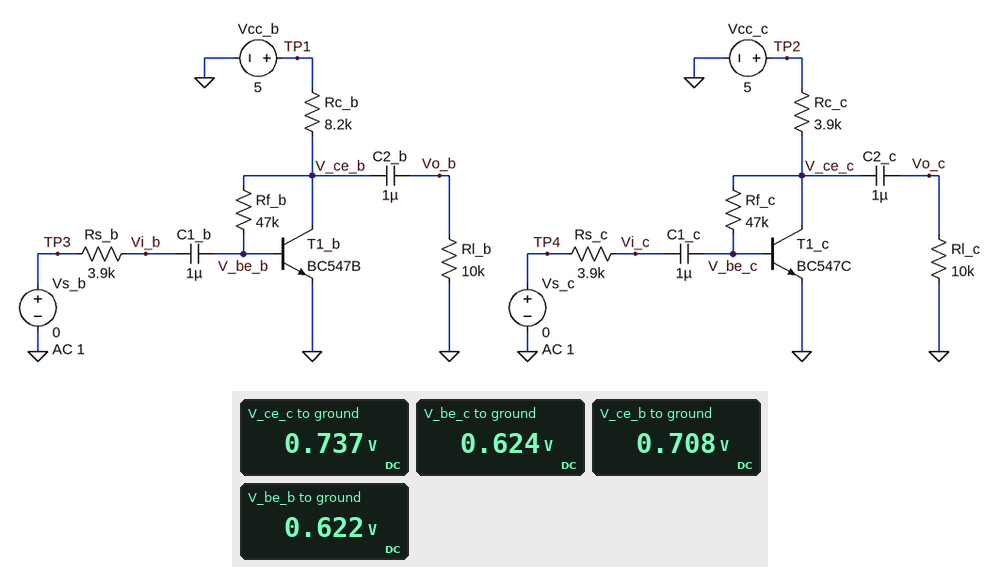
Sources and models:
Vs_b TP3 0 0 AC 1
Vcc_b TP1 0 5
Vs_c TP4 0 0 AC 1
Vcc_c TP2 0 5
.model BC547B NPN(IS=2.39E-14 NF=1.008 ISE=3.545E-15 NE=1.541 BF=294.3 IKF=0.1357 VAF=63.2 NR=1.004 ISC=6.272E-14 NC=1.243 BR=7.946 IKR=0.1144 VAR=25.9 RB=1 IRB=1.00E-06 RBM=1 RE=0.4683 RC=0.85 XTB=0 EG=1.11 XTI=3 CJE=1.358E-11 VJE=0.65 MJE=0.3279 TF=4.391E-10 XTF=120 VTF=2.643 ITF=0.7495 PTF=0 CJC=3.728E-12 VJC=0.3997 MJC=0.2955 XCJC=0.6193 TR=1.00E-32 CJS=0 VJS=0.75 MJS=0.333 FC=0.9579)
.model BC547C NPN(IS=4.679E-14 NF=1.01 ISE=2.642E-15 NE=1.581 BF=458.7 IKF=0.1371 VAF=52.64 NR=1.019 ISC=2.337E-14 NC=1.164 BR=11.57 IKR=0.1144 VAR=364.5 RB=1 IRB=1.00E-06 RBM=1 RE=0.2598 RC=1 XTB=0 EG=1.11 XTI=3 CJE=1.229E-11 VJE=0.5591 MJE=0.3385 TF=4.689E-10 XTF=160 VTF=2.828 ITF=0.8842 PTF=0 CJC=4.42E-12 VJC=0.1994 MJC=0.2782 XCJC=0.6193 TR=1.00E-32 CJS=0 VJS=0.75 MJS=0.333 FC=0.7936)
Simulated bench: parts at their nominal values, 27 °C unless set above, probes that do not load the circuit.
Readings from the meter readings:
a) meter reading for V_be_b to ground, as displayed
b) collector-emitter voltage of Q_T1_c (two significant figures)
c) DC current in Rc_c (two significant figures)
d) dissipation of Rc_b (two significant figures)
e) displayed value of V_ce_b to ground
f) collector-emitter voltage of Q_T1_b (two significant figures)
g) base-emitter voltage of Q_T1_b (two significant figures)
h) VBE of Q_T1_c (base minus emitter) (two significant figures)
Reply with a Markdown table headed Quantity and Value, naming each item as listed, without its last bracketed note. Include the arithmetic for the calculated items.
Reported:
| Quantity | Value |
|---|---|
| meter reading for V_be_b to ground, as displayed | 0.622 V |
| collector-emitter voltage of Q_T1_c | 737 mV = 740 mV |
| DC current in Rc_c | (5 V - 737 mV) / 3.9 kΩ = 1.1 mA |
| dissipation of Rc_b | (5 V - 708 mV)^2 / 8.2 kΩ = 2.2 mW |
| displayed value of V_ce_b to ground | 0.708 V |
| collector-emitter voltage of Q_T1_b | 708 mV = 710 mV |
| base-emitter voltage of Q_T1_b | 622 mV = 620 mV |
| VBE of Q_T1_c (base minus emitter) | 624 mV = 620 mV |
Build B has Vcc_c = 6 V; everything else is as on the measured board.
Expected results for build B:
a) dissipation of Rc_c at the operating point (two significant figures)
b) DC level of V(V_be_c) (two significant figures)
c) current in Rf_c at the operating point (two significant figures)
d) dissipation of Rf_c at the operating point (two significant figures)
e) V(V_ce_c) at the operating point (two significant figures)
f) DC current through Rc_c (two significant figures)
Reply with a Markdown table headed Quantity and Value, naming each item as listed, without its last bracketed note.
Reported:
| Quantity | Value |
|---|---|
| dissipation of Rc_c at the operating point | 7.0 mW |
| DC level of V(V_be_c) | 630 mV |
| current in Rf_c at the operating point | 3.0 µA |
| dissipation of Rf_c at the operating point | 410 nW |
| V(V_ce_c) at the operating point | 770 mV |
| DC current through Rc_c | 1.3 mA |
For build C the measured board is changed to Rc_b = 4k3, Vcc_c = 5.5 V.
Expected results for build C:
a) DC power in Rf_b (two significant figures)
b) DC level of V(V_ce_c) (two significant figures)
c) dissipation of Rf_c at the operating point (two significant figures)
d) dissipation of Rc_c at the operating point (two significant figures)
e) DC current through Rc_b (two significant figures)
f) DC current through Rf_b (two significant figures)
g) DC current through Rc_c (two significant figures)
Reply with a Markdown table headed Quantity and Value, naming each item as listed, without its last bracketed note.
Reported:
| Quantity | Value |
|---|---|
| DC power in Rf_b | 560 nW |
| DC level of V(V_ce_c) | 750 mV |
| dissipation of Rf_c at the operating point | 340 nW |
| dissipation of Rc_c at the operating point | 5.8 mW |
| DC current through Rc_b | 980 µA |
| DC current through Rf_b | 3.4 µA |
| DC current through Rc_c | 1.2 mA |
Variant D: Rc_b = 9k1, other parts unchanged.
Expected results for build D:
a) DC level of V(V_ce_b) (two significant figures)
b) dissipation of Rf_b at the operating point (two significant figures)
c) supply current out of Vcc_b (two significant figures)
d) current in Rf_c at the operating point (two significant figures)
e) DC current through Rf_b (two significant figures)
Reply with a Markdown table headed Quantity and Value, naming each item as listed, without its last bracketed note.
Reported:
| Quantity | Value |
|---|---|
| DC level of V(V_ce_b) | 700 mV |
| dissipation of Rf_b at the operating point | 130 nW |
| supply current out of Vcc_b | 470 µA |
| current in Rf_c at the operating point | 2.4 µA |
| DC current through Rf_b | 1.7 µA |
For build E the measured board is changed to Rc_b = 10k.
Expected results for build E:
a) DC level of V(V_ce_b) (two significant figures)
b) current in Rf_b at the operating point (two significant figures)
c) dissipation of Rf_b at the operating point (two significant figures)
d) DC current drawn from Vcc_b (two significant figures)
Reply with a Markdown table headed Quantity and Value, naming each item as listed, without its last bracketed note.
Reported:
| Quantity | Value |
|---|---|
| DC level of V(V_ce_b) | 690 mV |
| current in Rf_b at the operating point | 1.5 µA |
| dissipation of Rf_b at the operating point | 110 nW |
| DC current drawn from Vcc_b | 430 µA |
